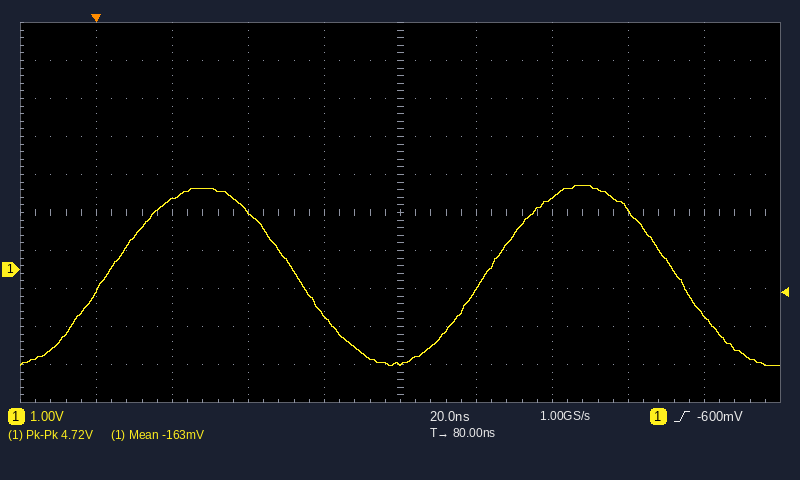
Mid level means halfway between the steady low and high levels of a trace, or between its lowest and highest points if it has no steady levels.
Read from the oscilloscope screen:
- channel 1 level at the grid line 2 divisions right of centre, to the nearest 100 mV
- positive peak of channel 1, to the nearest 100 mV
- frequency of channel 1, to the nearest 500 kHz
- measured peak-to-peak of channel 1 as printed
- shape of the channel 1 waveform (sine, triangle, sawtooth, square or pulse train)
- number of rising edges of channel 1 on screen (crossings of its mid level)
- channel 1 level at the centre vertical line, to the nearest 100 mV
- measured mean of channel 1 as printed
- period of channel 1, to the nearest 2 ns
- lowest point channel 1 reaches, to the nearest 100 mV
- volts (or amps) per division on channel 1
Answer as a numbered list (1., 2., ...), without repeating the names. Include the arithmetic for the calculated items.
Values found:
1. 1.9 V
2. 2.2 V
3. 1 / 100 ns ≈ 10.0 MHz
4. 4.72 V
5. sine
6. 2
7. -2.5 V
8. -163 mV
9. 100 ns
10. -2.5 V
11. 1 V
